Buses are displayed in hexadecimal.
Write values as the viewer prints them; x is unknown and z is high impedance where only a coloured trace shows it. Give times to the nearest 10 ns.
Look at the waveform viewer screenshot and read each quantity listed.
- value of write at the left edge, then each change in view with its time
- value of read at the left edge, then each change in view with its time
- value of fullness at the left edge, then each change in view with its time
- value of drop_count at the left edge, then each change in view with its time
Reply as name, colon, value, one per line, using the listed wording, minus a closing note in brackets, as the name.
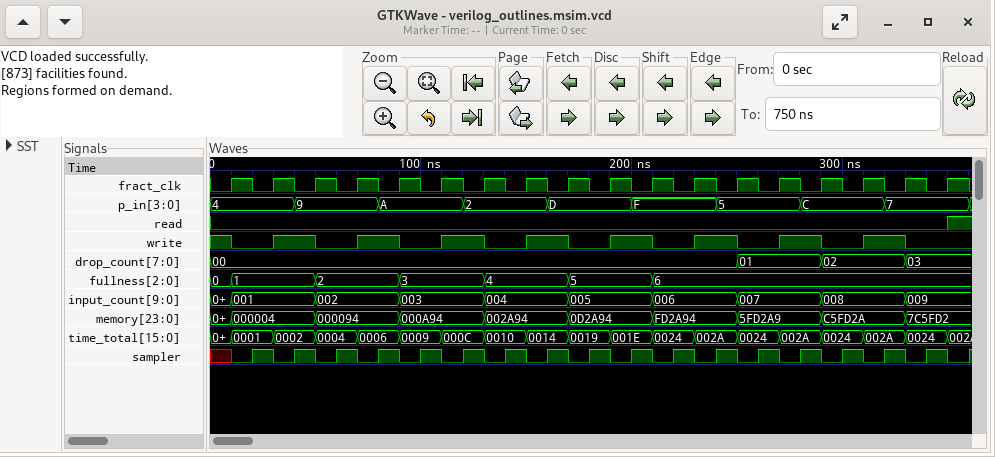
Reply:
value of write at the left edge, then each change in view with its time: 1, 0 at 10 ns, 1 at 30 ns, 0 at 50 ns, 1 at 70 ns, 0 at 90 ns, 1 at 110 ns, 0 at 130 ns, 1 at 150 ns, 0 at 170 ns, 1 at 190 ns, 0 at 210 ns, 1 at 230 ns, 0 at 250 ns, 1 at 270 ns, 0 at 290 ns, 1 at 310 ns, 0 at 330 ns
value of read at the left edge, then each change in view with its time: 0, 1 at 350 ns
value of fullness at the left edge, then each change in view with its time: 0, 1 at 10 ns, 2 at 50 ns, 3 at 90 ns, 4 at 130 ns, 5 at 170 ns, 6 at 210 ns
value of drop_count at the left edge, then each change in view with its time: 00, 01 at 250 ns, 02 at 290 ns, 03 at 330 ns
